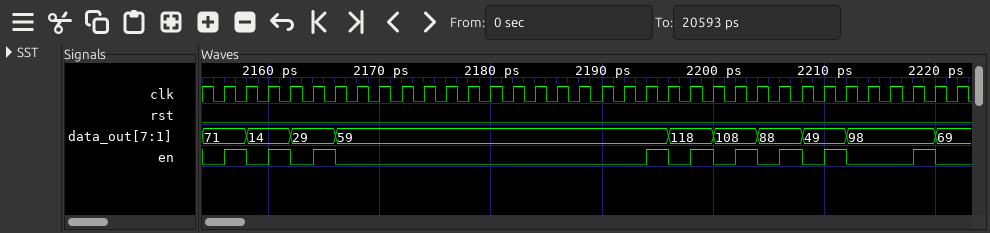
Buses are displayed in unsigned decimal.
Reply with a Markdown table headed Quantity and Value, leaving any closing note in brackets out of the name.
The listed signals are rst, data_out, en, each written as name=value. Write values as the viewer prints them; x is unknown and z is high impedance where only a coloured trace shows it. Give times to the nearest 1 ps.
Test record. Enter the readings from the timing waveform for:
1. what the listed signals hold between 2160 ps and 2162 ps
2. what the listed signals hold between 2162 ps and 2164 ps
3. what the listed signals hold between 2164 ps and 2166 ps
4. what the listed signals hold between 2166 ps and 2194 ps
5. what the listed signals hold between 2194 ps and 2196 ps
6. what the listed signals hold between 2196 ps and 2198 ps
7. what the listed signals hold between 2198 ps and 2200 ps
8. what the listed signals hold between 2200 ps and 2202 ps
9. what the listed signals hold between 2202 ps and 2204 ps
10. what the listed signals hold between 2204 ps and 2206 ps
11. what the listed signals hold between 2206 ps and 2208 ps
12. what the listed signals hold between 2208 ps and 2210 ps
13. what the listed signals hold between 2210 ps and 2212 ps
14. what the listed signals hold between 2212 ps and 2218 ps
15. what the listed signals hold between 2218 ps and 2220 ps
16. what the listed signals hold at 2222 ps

| Quantity | Value |
|---|---|
| what the listed signals hold between 2160 ps and 2162 ps | rst=0, data_out=14, en=1 |
| what the listed signals hold between 2162 ps and 2164 ps | rst=0, data_out=29, en=0 |
| what the listed signals hold between 2164 ps and 2166 ps | rst=0, data_out=29, en=1 |
| what the listed signals hold between 2166 ps and 2194 ps | rst=0, data_out=59, en=0 |
| what the listed signals hold between 2194 ps and 2196 ps | rst=0, data_out=59, en=1 |
| what the listed signals hold between 2196 ps and 2198 ps | rst=0, data_out=118, en=0 |
| what the listed signals hold between 2198 ps and 2200 ps | rst=0, data_out=118, en=1 |
| what the listed signals hold between 2200 ps and 2202 ps | rst=0, data_out=108, en=0 |
| what the listed signals hold between 2202 ps and 2204 ps | rst=0, data_out=108, en=1 |
| what the listed signals hold between 2204 ps and 2206 ps | rst=0, data_out=88, en=0 |
| what the listed signals hold between 2206 ps and 2208 ps | rst=0, data_out=88, en=1 |
| what the listed signals hold between 2208 ps and 2210 ps | rst=0, data_out=49, en=0 |
| what the listed signals hold between 2210 ps and 2212 ps | rst=0, data_out=49, en=1 |
| what the listed signals hold between 2212 ps and 2218 ps | rst=0, data_out=98, en=0 |
| what the listed signals hold between 2218 ps and 2220 ps | rst=0, data_out=98, en=1 |
| what the listed signals hold at 2222 ps | rst=0, data_out=69, en=0 |
